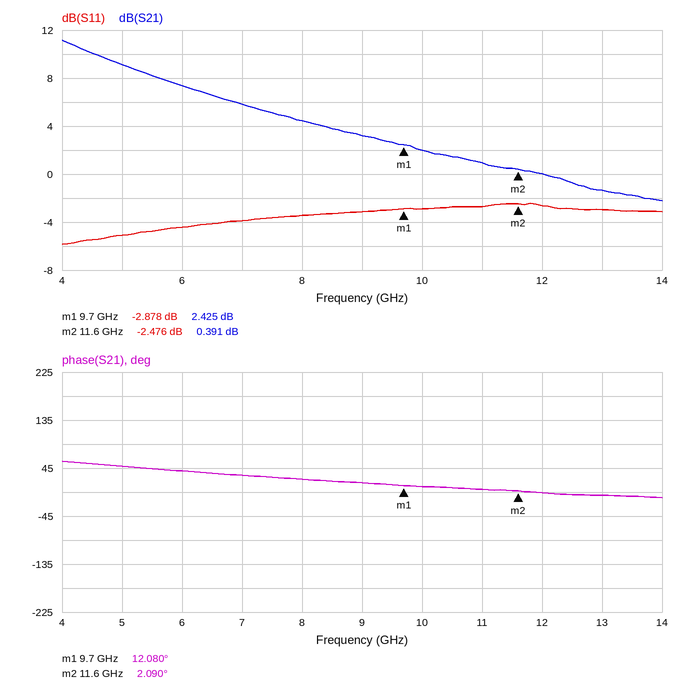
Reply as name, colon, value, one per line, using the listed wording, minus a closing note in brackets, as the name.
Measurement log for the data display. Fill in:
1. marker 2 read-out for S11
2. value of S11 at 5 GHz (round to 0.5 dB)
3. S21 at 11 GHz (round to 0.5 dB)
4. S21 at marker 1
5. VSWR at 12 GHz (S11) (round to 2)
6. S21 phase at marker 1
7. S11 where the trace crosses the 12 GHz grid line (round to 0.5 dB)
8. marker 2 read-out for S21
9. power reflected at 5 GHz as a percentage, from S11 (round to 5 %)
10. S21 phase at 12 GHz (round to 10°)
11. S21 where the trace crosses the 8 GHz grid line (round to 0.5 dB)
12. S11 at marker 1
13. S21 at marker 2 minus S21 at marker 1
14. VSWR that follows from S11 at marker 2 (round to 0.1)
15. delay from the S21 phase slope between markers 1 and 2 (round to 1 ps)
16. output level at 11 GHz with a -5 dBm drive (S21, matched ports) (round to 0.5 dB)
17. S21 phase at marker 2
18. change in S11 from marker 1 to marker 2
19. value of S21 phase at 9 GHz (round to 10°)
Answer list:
marker 2 read-out for S11: -2.476 dB
value of S11 at 5 GHz: -5.0 dB
S21 at 11 GHz: 1.0 dB
S21 at marker 1: 2.425 dB
VSWR at 12 GHz (S11): 6
S21 phase at marker 1: 12.080°
S11 where the trace crosses the 12 GHz grid line: -2.5 dB
marker 2 read-out for S21: 0.391 dB
power reflected at 5 GHz as a percentage, from S11: 30 %
S21 phase at 12 GHz: 0°
S21 where the trace crosses the 8 GHz grid line: 4.5 dB
S11 at marker 1: -2.878 dB
S21 at marker 2 minus S21 at marker 1: -2.034 dB
VSWR that follows from S11 at marker 2: 7.1
delay from the S21 phase slope between markers 1 and 2: 15 ps
output level at 11 GHz with a -5 dBm drive (S21, matched ports): -4.0 dBm
S21 phase at marker 2: 2.090°
change in S11 from marker 1 to marker 2: 0.402 dB
value of S21 phase at 9 GHz: 20°
